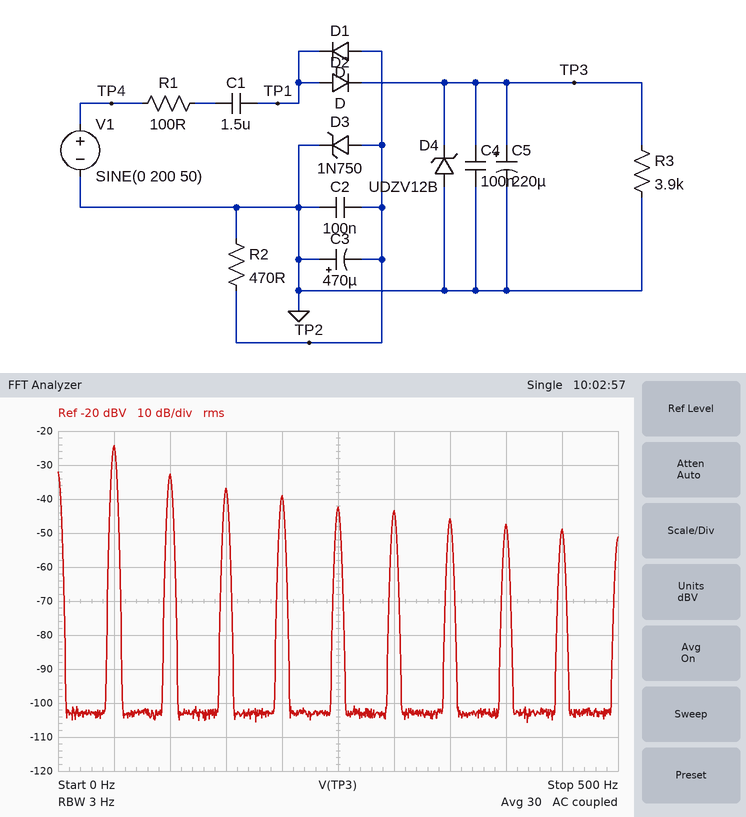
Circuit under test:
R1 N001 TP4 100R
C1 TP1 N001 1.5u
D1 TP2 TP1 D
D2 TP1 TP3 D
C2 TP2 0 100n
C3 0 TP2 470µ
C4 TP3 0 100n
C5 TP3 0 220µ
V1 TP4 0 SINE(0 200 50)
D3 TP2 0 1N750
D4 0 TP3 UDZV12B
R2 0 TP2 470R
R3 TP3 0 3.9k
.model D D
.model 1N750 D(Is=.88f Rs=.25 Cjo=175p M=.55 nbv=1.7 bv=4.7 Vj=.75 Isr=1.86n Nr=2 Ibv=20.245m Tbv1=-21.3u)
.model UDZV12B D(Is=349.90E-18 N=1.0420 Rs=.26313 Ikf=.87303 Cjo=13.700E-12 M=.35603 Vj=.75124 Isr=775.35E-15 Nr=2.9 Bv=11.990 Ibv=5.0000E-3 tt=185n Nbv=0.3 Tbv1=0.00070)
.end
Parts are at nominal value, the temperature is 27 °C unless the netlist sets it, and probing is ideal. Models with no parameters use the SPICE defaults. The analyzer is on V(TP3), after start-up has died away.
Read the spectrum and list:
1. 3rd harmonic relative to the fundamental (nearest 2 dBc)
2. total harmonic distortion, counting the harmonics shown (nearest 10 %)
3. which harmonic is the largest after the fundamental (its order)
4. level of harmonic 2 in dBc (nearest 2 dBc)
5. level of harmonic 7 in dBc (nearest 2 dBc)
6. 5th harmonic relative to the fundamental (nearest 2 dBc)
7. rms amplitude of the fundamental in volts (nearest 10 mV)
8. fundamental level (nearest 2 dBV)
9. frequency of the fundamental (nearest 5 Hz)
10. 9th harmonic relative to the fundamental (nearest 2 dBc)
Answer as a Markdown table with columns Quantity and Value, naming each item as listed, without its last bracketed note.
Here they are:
| Quantity | Value |
|---|---|
| 3rd harmonic relative to the fundamental | -12 dBc |
| total harmonic distortion, counting the harmonics shown | 50 % |
| which harmonic is the largest after the fundamental | 2 |
| level of harmonic 2 in dBc | -8 dBc |
| level of harmonic 7 in dBc | -22 dBc |
| 5th harmonic relative to the fundamental | -18 dBc |
| rms amplitude of the fundamental in volts | 60 mV |
| fundamental level | -24 dBV |
| frequency of the fundamental | 50 Hz |
| 9th harmonic relative to the fundamental | -24 dBc |
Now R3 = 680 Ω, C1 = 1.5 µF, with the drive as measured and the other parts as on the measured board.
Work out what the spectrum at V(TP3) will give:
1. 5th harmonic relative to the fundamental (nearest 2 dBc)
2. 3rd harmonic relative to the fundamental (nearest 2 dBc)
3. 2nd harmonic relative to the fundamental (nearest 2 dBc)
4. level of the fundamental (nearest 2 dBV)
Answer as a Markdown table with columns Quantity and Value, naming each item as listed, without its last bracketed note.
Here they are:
| Quantity | Value |
|---|---|
| 5th harmonic relative to the fundamental | -30 dBc |
| 3rd harmonic relative to the fundamental | -16 dBc |
| 2nd harmonic relative to the fundamental | -10 dBc |
| level of the fundamental | -10 dBV |
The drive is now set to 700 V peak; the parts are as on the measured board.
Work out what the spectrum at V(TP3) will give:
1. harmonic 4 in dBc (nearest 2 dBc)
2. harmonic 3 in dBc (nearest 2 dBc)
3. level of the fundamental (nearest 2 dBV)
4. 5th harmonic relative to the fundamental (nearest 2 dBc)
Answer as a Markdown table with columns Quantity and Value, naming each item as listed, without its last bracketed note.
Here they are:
| Quantity | Value |
|---|---|
| harmonic 4 in dBc | -16 dBc |
| harmonic 3 in dBc | -14 dBc |
| level of the fundamental | -22 dBV |
| 5th harmonic relative to the fundamental | -20 dBc |
